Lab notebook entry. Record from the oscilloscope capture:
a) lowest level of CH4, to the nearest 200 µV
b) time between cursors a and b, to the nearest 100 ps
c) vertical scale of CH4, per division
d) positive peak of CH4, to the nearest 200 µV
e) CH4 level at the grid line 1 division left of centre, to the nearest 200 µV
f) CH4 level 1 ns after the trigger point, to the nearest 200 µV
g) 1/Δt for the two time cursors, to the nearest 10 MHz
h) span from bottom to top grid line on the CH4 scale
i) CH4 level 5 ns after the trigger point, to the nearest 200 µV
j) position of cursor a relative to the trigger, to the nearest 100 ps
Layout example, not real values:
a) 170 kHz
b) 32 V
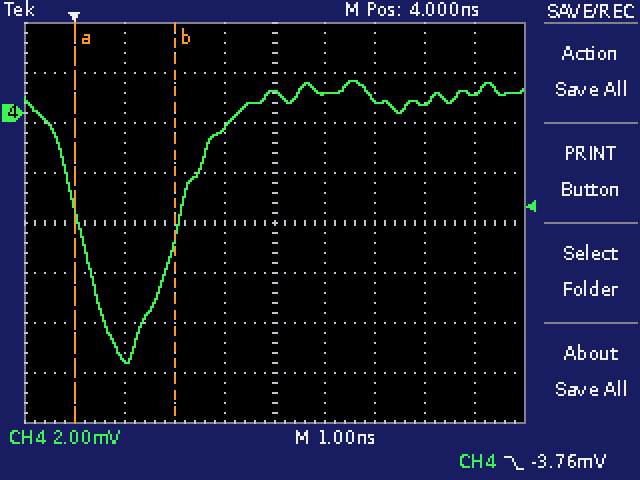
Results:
a) -10.0 mV
b) 2.0 ns
c) 2 mV
d) 1.2 mV
e) -600 µV
f) -9.8 mV
g) 500 MHz
h) 16 mV
i) 800 µV
j) 0.0 ns
